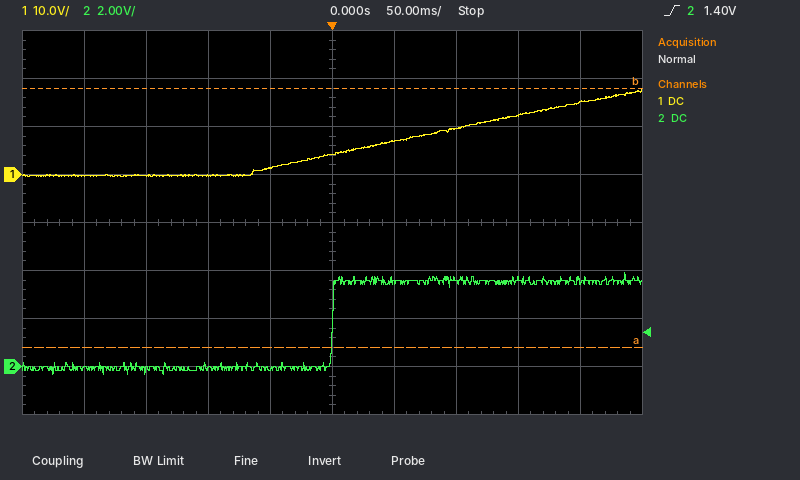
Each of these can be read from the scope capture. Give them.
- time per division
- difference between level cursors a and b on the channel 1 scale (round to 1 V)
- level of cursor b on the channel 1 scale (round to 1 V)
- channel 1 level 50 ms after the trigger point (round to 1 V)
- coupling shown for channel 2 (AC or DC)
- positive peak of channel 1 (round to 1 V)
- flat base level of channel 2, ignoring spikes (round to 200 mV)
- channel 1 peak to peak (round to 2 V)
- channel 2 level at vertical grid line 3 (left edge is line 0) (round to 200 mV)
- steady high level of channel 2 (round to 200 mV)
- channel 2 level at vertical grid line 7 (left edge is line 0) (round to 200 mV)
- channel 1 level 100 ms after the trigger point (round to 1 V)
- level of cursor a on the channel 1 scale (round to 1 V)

50 ms
54 V
18 V
7 V
DC
18 V
0.0 V
18 V
0.0 V
3.6 V
3.6 V
10 V
-36 V
